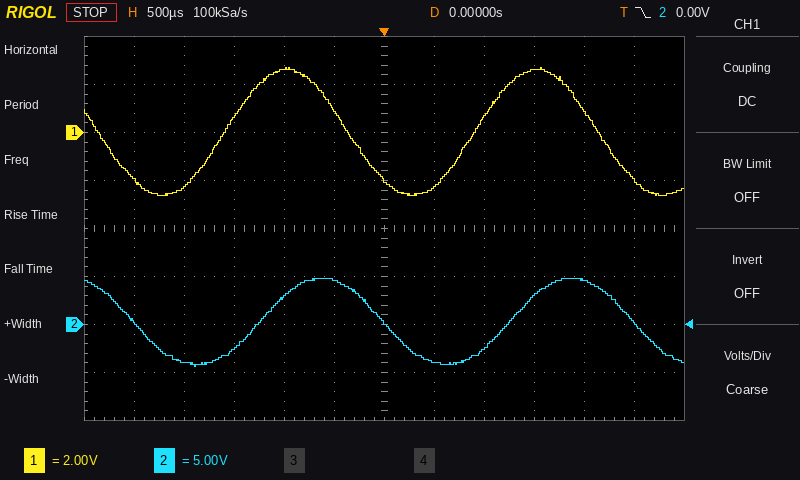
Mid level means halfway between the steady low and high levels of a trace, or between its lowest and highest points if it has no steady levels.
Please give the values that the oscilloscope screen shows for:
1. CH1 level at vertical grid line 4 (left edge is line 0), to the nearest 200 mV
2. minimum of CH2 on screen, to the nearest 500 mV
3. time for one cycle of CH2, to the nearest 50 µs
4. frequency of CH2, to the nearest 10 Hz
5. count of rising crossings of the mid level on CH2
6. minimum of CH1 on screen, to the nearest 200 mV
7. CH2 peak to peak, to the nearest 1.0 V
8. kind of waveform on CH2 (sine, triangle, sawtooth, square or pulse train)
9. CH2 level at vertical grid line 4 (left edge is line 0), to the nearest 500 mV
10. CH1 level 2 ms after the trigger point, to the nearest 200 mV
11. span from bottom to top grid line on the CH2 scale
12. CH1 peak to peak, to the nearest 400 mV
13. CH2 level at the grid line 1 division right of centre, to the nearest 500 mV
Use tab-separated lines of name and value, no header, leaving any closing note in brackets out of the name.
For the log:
CH1 level at vertical grid line 4 (left edge is line 0), to the nearest 200 mV	2.6 V
minimum of CH2 on screen, to the nearest 500 mV	-4.5 V
time for one cycle of CH2, to the nearest 50 µs	2.50 ms
frequency of CH2, to the nearest 10 Hz	400 Hz
count of rising crossings of the mid level on CH2	2
minimum of CH1 on screen, to the nearest 200 mV	-2.6 V
CH2 peak to peak, to the nearest 1.0 V	9.0 V
kind of waveform on CH2	sine
CH2 level at vertical grid line 4 (left edge is line 0), to the nearest 500 mV	3.0 V
CH1 level 2 ms after the trigger point, to the nearest 200 mV	800 mV
span from bottom to top grid line on the CH2 scale	40 V
CH1 peak to peak, to the nearest 400 mV	5.2 V
CH2 level at the grid line 1 division right of centre, to the nearest 500 mV	-4.0 V
